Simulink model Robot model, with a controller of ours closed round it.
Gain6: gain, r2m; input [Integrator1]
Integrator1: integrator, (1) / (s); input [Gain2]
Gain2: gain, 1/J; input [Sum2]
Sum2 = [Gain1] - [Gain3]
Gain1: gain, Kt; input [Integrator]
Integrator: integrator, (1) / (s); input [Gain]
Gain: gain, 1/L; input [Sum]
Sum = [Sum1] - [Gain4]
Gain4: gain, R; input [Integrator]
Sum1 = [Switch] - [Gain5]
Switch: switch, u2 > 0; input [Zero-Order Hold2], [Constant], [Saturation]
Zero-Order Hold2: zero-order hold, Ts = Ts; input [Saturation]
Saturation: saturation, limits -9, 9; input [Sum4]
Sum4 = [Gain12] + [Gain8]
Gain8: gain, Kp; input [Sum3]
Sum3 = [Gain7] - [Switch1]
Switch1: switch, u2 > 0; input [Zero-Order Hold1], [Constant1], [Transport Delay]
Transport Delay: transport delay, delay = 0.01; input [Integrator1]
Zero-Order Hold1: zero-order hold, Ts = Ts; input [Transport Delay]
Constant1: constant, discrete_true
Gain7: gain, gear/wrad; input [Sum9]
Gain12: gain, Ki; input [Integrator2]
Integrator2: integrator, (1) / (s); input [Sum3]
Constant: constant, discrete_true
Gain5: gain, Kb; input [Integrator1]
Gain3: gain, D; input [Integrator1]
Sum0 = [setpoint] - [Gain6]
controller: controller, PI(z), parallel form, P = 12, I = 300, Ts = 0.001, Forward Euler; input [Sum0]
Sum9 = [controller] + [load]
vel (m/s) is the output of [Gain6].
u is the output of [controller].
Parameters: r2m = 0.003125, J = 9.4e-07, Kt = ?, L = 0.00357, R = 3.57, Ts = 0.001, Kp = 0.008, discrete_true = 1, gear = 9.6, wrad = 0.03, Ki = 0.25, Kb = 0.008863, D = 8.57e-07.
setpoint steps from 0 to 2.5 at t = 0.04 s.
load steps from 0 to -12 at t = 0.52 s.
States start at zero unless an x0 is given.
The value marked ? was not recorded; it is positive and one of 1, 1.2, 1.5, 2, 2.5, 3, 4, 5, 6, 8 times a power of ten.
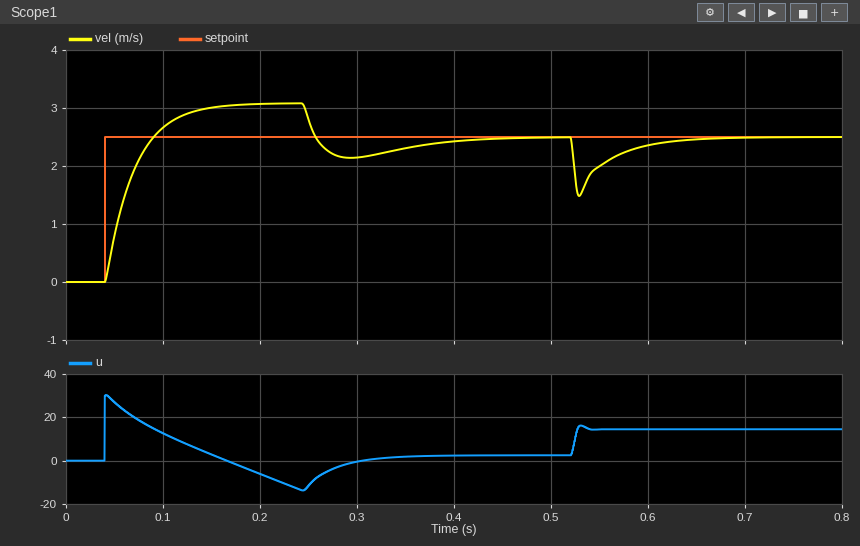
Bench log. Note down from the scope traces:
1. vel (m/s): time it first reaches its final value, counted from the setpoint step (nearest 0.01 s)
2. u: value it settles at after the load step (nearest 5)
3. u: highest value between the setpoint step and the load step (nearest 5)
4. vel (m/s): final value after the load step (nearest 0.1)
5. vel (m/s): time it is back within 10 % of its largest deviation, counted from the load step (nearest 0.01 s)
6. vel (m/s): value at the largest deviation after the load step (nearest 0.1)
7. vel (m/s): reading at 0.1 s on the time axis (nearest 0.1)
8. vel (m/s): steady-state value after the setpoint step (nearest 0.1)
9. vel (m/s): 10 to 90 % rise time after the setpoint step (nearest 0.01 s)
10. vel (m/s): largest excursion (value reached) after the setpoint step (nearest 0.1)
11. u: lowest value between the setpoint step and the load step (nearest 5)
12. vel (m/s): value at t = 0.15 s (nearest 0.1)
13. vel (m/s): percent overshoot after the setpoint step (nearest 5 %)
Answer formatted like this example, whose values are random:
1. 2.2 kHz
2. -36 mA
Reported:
1. 0.05 s
2. 15
3. 30
4. 2.5
5. 0.09 s
6. 1.5
7. 2.7
8. 2.5
9. 0.04 s
10. 3.1
11. -15
12. 3.0
13. 25 %
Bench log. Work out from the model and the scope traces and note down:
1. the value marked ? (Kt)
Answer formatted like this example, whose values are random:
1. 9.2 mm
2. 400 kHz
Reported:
1. 0.012
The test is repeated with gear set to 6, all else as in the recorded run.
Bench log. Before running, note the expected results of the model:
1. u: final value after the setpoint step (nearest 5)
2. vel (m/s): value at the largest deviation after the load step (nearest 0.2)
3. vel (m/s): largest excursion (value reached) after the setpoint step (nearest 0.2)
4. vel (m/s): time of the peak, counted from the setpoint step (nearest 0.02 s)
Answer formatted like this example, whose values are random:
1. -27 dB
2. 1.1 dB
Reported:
1. 5
2. 1.6
3. 3.0
4. 0.18 s
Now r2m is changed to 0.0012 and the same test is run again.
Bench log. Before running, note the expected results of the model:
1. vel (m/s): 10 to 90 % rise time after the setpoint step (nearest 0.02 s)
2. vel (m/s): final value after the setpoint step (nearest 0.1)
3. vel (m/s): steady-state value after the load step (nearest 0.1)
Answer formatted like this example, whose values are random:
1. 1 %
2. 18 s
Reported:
1. 0.06 s
2. 1.2
3. 1.2
